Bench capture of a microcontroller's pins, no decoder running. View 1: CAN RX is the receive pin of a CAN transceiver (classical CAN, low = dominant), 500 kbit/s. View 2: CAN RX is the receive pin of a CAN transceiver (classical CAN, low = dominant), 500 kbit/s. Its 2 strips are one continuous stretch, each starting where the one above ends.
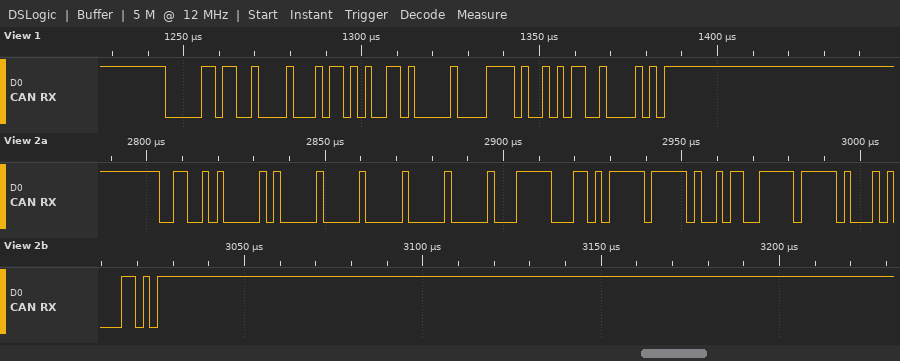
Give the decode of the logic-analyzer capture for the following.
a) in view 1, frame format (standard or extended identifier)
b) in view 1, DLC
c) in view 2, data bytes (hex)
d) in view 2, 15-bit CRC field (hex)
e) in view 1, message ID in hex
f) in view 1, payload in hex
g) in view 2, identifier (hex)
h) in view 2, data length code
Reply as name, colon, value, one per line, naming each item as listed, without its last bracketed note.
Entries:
in view 1, frame format: standard
in view 1, DLC: 4
in view 2, data bytes: 00 00 00 7C D7 FF 2C FF
in view 2, 15-bit CRC field: 0x7146
in view 1, message ID in hex: 0x059
in view 1, payload in hex: 5A 9A 00 F4
in view 2, identifier: 0x328
in view 2, data length code: 8
